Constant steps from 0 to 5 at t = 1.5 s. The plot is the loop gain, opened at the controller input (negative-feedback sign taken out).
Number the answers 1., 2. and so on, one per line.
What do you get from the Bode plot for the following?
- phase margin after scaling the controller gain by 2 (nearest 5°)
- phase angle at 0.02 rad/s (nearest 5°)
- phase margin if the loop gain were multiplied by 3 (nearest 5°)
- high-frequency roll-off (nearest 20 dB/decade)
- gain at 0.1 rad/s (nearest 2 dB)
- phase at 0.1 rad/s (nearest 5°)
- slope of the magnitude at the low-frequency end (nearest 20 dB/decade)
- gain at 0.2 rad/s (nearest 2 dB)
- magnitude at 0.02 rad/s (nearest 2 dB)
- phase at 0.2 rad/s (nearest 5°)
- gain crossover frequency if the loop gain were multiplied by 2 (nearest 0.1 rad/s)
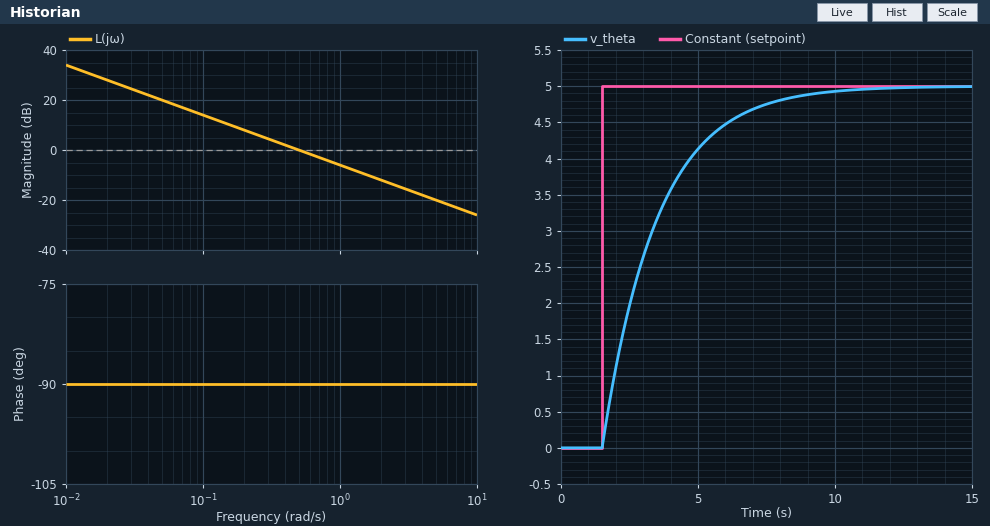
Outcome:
1. 90°
2. -90°
3. 90°
4. -20 dB/decade
5. 14 dB
6. -90°
7. -20 dB/decade
8. 8 dB
9. 28 dB
10. -90°
11. 1.0 rad/s
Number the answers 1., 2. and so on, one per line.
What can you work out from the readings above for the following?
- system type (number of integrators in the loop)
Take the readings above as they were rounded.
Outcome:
1. 1
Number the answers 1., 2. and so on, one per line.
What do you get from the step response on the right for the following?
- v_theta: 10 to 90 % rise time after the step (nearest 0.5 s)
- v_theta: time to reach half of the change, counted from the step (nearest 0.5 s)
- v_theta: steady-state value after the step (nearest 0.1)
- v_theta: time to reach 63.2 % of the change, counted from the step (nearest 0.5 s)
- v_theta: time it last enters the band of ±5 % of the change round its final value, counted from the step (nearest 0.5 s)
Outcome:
1. 4.5 s
2. 1.5 s
3. 5.0
4. 2.0 s
5. 6.0 s
